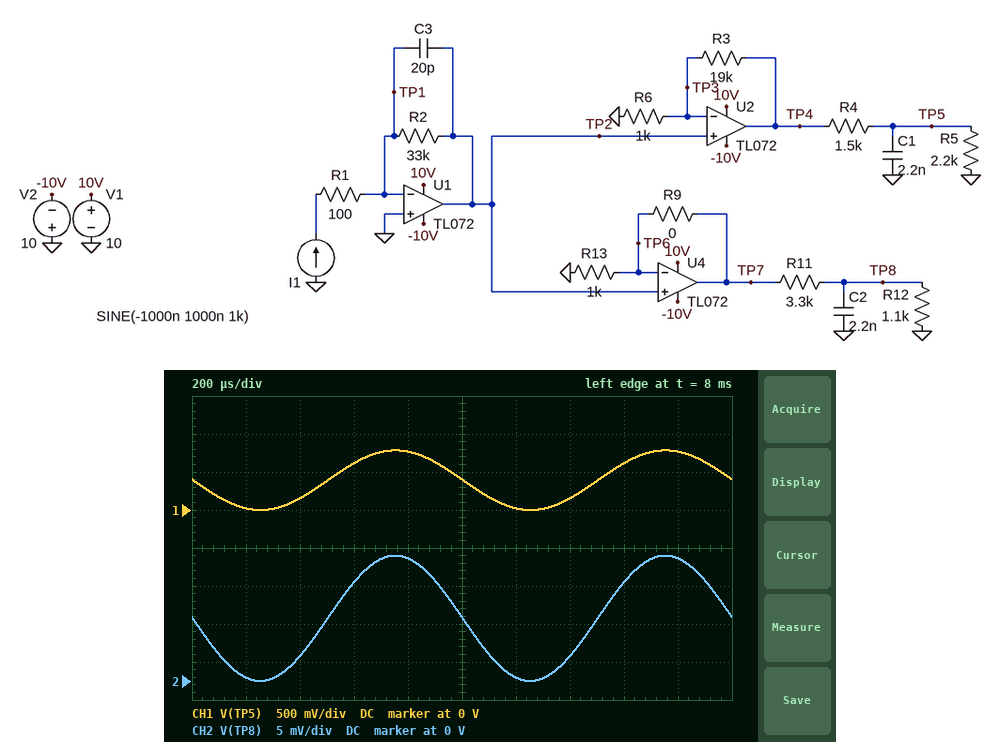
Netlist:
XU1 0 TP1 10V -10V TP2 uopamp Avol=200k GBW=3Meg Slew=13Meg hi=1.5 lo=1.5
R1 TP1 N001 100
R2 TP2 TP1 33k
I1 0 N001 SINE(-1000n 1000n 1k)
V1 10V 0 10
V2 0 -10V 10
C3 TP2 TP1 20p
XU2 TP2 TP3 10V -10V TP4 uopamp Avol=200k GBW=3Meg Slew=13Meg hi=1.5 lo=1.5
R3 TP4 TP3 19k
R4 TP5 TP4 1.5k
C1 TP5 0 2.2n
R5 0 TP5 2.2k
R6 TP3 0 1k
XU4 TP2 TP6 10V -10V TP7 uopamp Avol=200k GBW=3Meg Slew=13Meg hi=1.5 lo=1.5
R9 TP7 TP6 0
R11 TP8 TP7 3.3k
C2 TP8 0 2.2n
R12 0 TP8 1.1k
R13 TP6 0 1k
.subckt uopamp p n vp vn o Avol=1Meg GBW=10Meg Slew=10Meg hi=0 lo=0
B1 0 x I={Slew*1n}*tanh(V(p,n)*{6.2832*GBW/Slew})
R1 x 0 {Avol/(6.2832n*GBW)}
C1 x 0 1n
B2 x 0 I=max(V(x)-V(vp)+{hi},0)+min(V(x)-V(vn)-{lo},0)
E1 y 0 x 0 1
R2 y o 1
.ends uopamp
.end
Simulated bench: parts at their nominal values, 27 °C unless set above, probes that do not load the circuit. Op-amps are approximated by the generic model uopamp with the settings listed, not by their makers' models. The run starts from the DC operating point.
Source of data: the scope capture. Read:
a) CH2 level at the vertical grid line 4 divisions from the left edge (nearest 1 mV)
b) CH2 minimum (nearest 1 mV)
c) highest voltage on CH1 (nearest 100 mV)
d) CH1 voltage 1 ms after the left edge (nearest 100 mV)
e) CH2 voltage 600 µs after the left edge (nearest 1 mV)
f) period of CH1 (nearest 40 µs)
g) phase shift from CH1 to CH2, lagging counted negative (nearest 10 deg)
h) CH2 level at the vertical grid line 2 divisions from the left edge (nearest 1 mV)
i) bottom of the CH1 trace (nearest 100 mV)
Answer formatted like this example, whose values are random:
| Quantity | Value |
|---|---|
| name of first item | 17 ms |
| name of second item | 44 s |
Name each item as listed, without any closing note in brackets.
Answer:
| Quantity | Value |
|---|---|
| CH2 level at the vertical grid line 4 divisions from the left edge | 16 mV |
| CH2 minimum | 0 V |
| highest voltage on CH1 | 800 mV |
| CH1 voltage 1 ms after the left edge | 400 mV |
| CH2 voltage 600 µs after the left edge | 13 mV |
| period of CH1 | 1.00 ms |
| phase shift from CH1 to CH2, lagging counted negative | 0 deg |
| CH2 level at the vertical grid line 2 divisions from the left edge | 3 mV |
| bottom of the CH1 trace | 0 V |
